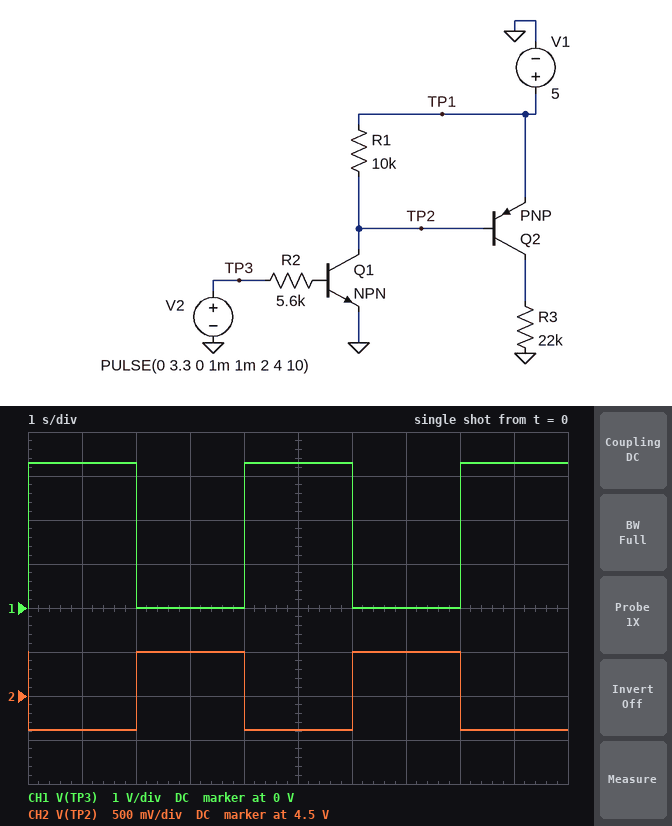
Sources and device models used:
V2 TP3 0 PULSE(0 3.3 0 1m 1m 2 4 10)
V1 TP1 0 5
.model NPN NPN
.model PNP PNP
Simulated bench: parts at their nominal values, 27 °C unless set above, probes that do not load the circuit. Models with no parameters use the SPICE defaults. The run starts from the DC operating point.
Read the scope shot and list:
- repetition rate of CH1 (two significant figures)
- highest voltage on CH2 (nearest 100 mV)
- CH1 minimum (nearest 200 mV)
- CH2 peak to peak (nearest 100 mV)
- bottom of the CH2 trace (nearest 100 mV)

250 mHz
5.0 V
0 V
900 mV
4.1 V
